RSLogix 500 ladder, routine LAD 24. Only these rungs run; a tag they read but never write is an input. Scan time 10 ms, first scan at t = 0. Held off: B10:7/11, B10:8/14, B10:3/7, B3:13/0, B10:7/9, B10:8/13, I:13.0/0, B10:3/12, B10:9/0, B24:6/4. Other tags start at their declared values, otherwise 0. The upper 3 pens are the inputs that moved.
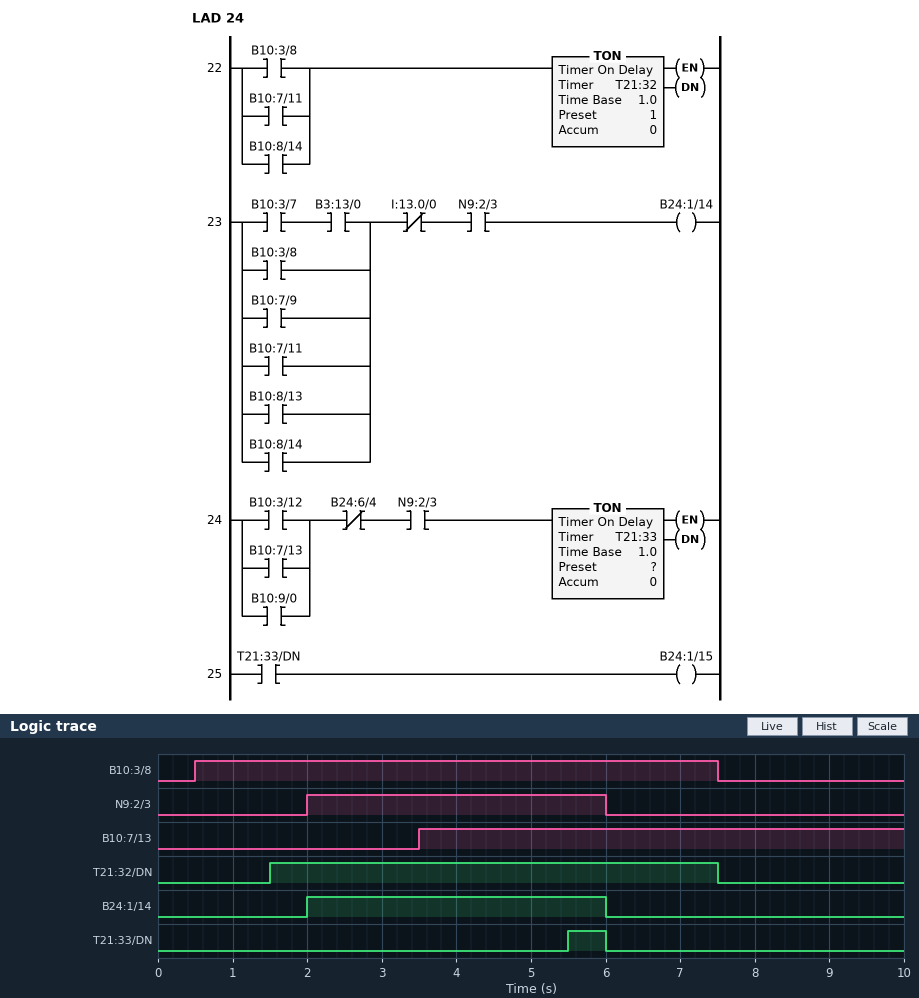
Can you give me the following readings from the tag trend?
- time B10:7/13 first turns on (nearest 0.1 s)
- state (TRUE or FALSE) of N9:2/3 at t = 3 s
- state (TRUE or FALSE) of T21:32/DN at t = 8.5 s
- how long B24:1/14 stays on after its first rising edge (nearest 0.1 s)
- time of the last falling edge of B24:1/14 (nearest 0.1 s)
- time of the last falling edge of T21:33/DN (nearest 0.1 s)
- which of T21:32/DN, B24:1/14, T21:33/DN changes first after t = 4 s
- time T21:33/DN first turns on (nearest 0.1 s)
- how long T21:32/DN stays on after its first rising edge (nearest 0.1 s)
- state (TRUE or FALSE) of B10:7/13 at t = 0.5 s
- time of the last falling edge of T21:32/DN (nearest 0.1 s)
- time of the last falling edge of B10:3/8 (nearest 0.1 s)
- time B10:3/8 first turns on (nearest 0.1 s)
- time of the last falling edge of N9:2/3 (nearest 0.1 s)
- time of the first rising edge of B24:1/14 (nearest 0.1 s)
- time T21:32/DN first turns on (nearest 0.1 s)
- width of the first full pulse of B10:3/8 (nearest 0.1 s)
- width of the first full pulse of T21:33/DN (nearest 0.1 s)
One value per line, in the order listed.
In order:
3.5 s
TRUE
FALSE
4.0 s
6.0 s
6.0 s
T21:33/DN
5.5 s
6.0 s
FALSE
7.5 s
7.5 s
0.5 s
6.0 s
2.0 s
1.5 s
7.0 s
0.5 s
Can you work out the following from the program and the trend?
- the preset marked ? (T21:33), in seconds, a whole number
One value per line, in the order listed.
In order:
2 s
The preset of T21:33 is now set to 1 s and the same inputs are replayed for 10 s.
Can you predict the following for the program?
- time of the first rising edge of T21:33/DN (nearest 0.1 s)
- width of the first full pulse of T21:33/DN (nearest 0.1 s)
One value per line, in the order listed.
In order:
4.5 s
1.5 s
